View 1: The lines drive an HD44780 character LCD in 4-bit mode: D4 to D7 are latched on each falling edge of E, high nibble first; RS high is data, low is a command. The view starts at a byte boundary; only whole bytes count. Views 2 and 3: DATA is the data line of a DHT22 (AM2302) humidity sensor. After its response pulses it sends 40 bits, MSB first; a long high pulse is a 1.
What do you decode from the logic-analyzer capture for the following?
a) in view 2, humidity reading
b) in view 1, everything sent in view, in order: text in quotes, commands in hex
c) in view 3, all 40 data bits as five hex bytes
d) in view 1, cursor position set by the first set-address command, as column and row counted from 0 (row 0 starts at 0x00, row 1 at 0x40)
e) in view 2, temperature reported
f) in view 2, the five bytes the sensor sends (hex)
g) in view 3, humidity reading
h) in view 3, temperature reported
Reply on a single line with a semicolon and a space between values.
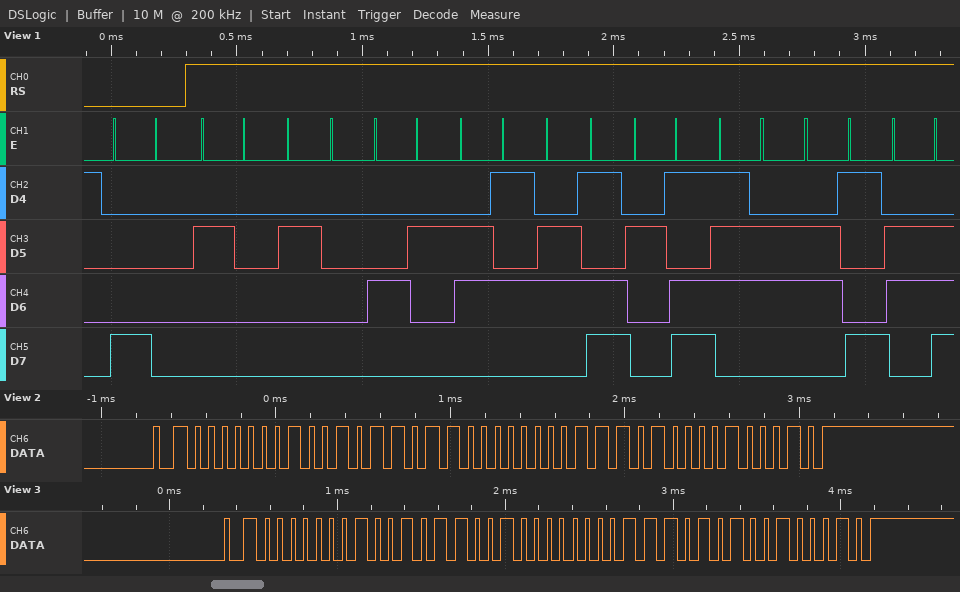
30.1 %; 0x80 "  Bem-vin"; 01 2C 80 75 22; column 0, row 0; -11.6 °C; 01 2D 80 74 22; 30.0 %; -11.7 °C
